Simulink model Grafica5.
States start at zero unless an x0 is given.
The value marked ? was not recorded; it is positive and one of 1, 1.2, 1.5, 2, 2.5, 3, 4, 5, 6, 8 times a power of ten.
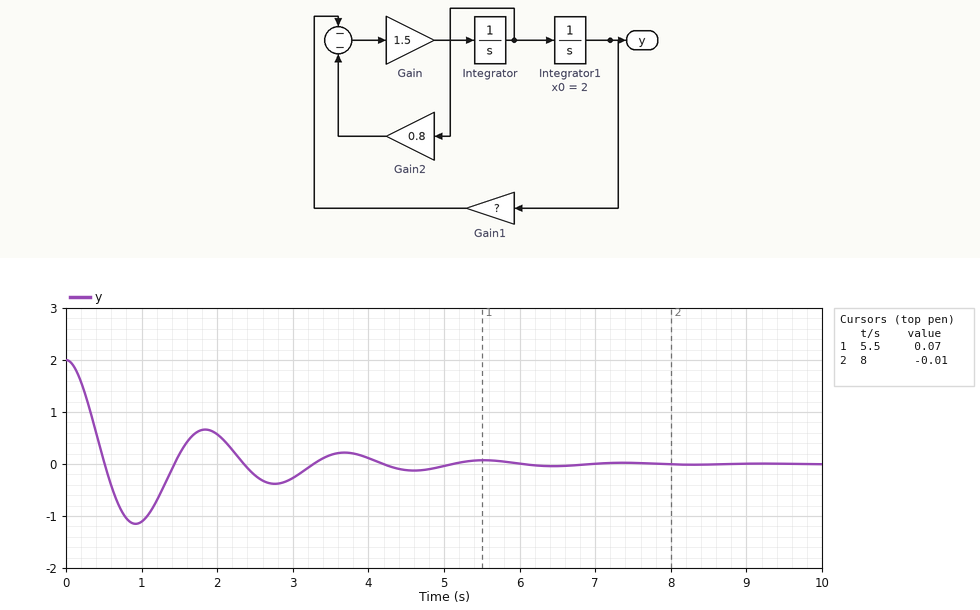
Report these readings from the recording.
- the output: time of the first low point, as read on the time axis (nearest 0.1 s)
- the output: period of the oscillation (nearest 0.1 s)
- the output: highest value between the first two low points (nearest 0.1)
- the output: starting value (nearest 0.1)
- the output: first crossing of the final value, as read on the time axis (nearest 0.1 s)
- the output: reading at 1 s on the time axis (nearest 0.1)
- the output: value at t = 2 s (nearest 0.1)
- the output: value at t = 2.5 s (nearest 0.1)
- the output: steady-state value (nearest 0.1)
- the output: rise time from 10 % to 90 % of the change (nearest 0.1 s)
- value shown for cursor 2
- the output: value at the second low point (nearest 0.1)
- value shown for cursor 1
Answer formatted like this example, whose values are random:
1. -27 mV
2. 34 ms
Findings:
1. 0.9 s
2. 1.8 s
3. 0.7
4. 2.0
5. 0.5 s
6. -1.1
7. 0.6
8. -0.2
9. 0.0
10. 0.3 s
11. -0.01
12. -0.4
13. 0.07
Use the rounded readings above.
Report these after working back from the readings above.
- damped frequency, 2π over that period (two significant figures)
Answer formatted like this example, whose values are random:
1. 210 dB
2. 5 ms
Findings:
1. 3.5 rad/s
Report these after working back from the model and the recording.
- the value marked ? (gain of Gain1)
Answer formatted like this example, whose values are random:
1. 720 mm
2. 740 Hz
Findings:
1. 8
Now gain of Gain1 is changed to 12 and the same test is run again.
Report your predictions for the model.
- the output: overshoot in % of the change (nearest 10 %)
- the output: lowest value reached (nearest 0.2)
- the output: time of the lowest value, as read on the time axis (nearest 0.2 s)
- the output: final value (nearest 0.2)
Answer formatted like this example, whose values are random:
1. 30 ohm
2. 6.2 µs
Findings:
1. 60 %
2. -1.2
3. 0.8 s
4. 0.0
